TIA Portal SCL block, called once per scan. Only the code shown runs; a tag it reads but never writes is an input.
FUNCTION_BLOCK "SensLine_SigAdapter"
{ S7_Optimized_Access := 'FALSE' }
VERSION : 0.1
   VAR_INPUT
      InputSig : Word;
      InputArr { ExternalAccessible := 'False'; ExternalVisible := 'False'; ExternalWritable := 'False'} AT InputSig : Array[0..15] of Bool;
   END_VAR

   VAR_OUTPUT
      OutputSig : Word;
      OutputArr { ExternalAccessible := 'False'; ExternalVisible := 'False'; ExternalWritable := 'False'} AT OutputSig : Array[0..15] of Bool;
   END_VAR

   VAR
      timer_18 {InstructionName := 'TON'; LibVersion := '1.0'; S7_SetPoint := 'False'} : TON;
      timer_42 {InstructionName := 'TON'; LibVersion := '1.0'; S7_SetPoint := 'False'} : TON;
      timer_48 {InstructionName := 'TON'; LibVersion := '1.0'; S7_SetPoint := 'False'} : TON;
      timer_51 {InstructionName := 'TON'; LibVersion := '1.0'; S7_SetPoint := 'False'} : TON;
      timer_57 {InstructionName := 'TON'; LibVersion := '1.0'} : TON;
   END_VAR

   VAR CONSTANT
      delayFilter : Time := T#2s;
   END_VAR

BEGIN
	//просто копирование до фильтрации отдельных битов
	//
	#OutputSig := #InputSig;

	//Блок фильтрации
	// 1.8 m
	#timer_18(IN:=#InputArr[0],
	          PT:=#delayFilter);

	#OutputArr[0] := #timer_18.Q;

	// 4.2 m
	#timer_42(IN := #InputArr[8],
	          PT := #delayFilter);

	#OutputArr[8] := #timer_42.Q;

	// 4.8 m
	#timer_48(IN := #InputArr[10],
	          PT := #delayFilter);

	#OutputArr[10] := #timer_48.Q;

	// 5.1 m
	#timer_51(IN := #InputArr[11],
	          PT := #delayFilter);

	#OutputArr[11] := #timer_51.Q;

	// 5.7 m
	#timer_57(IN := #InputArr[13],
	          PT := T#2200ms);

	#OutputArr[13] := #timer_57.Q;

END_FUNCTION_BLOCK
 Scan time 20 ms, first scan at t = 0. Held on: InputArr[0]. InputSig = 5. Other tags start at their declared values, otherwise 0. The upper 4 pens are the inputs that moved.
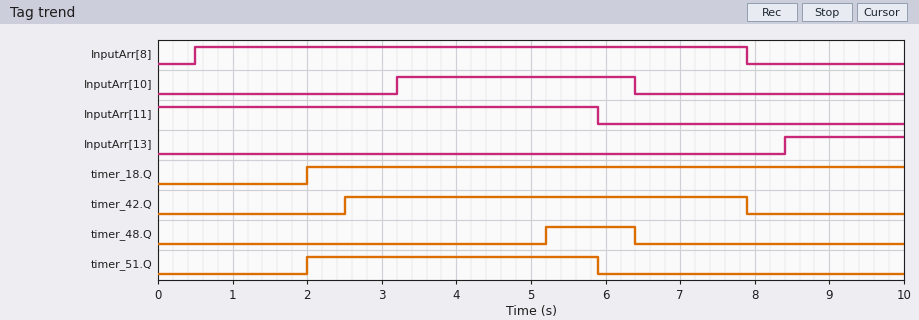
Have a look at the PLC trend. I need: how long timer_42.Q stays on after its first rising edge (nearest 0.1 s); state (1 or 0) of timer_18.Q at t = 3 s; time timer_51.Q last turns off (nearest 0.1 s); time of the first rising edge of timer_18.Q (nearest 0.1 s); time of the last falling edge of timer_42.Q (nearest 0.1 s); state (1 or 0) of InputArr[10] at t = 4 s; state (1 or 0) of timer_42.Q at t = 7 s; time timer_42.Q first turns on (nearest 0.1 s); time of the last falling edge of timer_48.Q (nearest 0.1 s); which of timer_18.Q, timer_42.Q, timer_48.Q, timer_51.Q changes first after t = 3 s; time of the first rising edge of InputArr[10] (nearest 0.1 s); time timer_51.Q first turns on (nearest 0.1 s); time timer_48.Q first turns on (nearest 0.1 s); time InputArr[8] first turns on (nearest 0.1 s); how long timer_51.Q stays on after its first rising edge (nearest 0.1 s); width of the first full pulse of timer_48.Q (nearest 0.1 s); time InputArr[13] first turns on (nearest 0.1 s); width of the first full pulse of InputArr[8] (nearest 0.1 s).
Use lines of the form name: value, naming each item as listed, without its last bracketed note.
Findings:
how long timer_42.Q stays on after its first rising edge: 5.4 s
state (1 or 0) of timer_18.Q at t = 3 s: 1
time timer_51.Q last turns off: 5.9 s
time of the first rising edge of timer_18.Q: 2.0 s
time of the last falling edge of timer_42.Q: 7.9 s
state (1 or 0) of InputArr[10] at t = 4 s: 1
state (1 or 0) of timer_42.Q at t = 7 s: 1
time timer_42.Q first turns on: 2.5 s
time of the last falling edge of timer_48.Q: 6.4 s
which of timer_18.Q, timer_42.Q, timer_48.Q, timer_51.Q changes first after t = 3 s: timer_48.Q
time of the first rising edge of InputArr[10]: 3.2 s
time timer_51.Q first turns on: 2.0 s
time timer_48.Q first turns on: 5.2 s
time InputArr[8] first turns on: 0.5 s
how long timer_51.Q stays on after its first rising edge: 3.9 s
width of the first full pulse of timer_48.Q: 1.2 s
time InputArr[13] first turns on: 8.4 s
width of the first full pulse of InputArr[8]: 7.4 s
